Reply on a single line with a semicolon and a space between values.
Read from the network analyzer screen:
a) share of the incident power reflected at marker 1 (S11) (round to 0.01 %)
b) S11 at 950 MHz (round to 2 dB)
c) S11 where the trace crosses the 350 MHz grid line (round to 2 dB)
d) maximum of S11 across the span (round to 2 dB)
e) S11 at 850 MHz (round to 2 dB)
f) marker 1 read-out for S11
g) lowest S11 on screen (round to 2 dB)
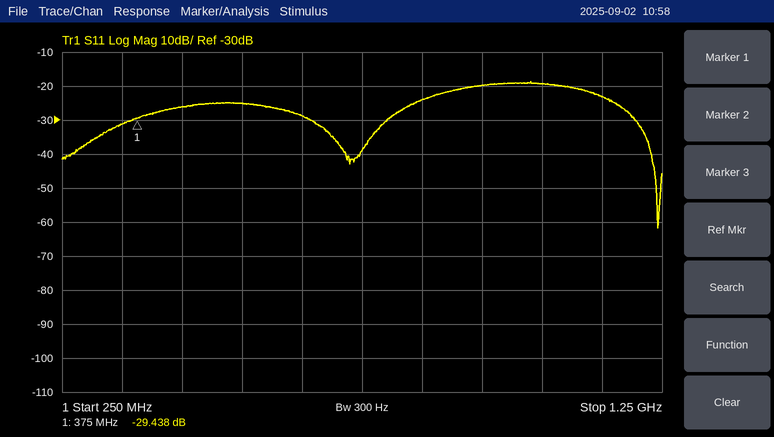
0.11 %; -20 dB; -32 dB; -18 dB; -24 dB; -29.438 dB; -62 dB
